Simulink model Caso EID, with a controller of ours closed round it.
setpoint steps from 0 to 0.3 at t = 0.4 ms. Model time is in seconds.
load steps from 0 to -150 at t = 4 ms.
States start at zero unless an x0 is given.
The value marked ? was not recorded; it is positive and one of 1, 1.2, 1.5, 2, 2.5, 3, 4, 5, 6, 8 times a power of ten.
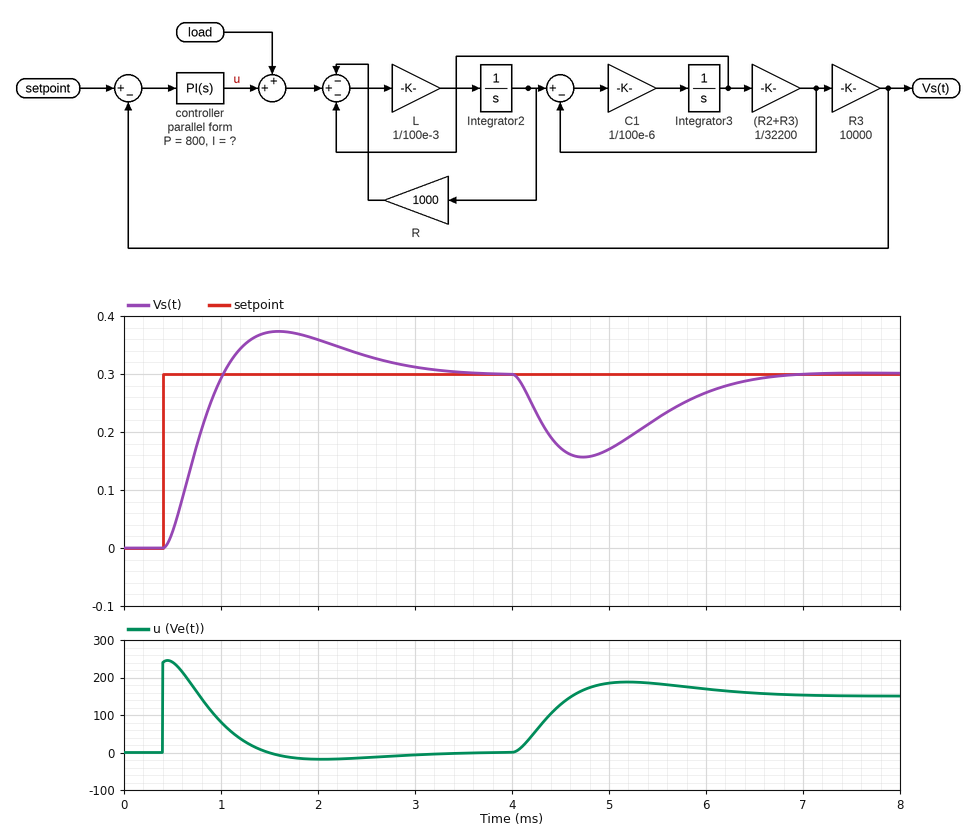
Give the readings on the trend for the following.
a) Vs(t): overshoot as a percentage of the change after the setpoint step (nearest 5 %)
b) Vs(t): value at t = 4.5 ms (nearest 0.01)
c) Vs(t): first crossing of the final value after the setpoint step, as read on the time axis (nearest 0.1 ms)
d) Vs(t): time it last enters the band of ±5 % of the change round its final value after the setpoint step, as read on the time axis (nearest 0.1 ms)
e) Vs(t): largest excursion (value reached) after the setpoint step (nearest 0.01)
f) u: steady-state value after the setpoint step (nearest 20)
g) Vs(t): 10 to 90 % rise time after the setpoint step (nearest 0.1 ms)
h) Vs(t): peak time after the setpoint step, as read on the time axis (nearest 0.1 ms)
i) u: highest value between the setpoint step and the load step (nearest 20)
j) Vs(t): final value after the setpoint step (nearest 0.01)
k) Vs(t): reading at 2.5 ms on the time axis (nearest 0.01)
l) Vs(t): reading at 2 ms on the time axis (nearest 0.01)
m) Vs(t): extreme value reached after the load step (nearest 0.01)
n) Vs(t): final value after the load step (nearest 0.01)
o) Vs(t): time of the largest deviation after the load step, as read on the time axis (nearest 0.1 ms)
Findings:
25 %
0.17
1.0 ms
2.9 ms
0.37
0
0.4 ms
1.6 ms
240
0.30
0.33
0.36
0.16
0.30
4.7 ms
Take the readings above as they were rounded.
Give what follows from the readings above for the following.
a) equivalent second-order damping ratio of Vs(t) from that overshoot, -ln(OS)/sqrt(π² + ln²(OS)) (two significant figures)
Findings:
0.40
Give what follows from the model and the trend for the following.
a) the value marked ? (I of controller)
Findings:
800000
